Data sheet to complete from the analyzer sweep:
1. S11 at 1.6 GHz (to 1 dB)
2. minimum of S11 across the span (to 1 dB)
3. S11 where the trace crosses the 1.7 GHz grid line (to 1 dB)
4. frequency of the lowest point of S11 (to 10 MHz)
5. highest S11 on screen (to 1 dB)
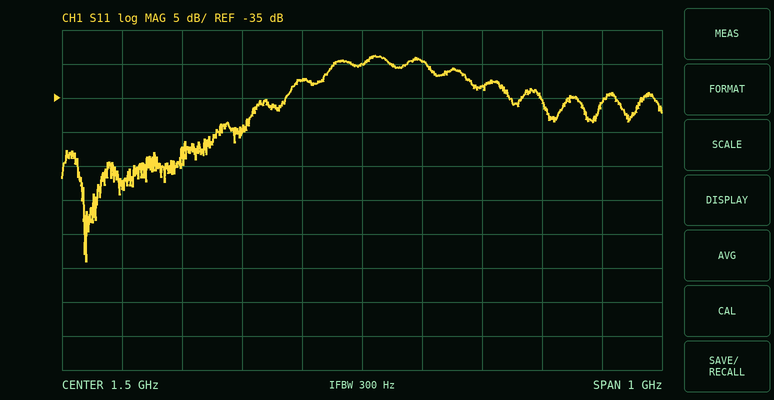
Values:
-30 dB
-59 dB
-33 dB
1.04 GHz
-29 dB
